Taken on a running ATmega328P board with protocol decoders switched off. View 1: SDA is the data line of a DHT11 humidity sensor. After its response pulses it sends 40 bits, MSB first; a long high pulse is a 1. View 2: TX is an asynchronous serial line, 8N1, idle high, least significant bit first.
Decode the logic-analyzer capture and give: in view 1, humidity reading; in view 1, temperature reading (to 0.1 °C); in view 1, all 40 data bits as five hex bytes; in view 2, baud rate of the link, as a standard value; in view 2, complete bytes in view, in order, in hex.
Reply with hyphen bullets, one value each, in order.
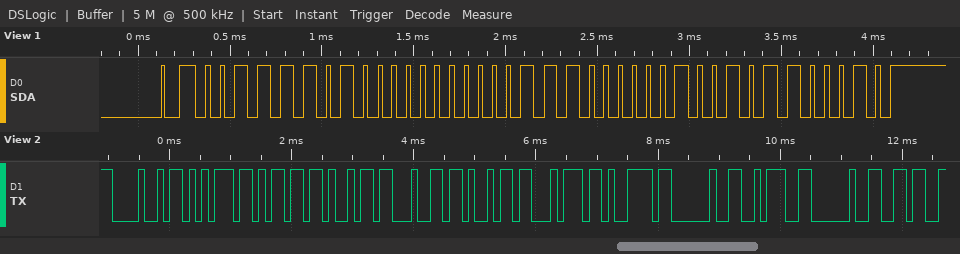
- 61 %
- 28.9 °C
- 3D 00 1C 09 62
- 9600 baud
- 0x48 0x75 0x6D 0x69 0x64 0x69 0x74 0x79 0x20 0x3A 0x20 0x36
